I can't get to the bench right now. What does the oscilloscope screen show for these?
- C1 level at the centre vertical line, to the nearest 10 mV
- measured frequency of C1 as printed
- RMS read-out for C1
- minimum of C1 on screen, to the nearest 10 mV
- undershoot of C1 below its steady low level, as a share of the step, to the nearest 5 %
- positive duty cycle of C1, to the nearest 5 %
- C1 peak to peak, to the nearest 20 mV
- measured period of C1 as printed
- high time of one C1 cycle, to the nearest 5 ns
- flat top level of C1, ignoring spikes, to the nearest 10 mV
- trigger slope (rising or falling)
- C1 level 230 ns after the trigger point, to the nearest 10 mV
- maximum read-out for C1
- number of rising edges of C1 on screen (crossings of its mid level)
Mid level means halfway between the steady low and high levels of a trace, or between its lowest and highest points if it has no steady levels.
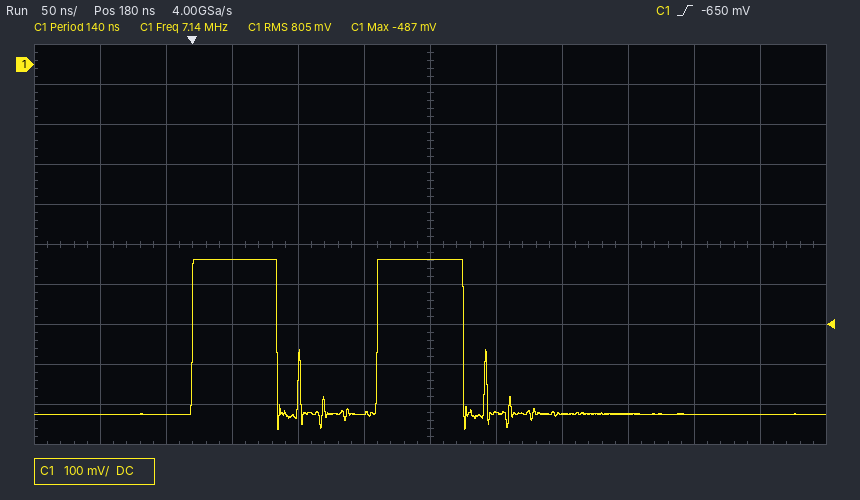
-490 mV
7.14 MHz
805 mV
-910 mV
10 %
45 %
420 mV
140 ns
65 ns
-490 mV
rising
-870 mV
-487 mV
2
